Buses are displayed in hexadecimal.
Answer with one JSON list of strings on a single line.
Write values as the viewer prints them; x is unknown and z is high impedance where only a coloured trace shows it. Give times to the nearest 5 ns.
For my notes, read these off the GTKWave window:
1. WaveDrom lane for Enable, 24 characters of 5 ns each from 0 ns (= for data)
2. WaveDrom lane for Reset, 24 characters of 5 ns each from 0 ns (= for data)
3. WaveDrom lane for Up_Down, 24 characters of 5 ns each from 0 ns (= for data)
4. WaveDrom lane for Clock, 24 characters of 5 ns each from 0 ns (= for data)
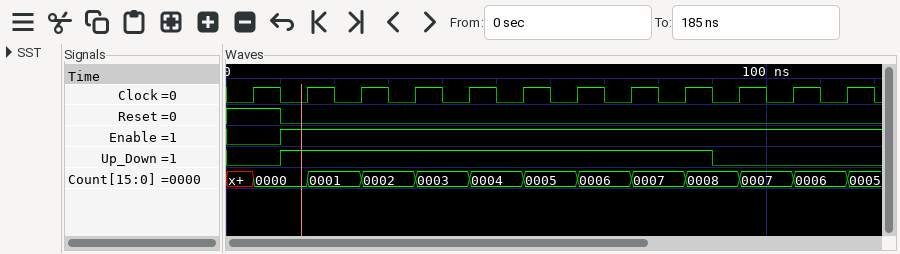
["{name: 'Enable', wave: '0.1.....................'}", "{name: 'Reset', wave: '1.0.....................'}", "{name: 'Up_Down', wave: '0.1...............0.....'}", "{name: 'Clock', wave: '010101010101010101010101'}"]
